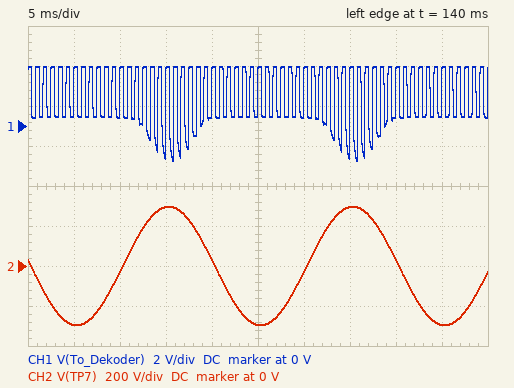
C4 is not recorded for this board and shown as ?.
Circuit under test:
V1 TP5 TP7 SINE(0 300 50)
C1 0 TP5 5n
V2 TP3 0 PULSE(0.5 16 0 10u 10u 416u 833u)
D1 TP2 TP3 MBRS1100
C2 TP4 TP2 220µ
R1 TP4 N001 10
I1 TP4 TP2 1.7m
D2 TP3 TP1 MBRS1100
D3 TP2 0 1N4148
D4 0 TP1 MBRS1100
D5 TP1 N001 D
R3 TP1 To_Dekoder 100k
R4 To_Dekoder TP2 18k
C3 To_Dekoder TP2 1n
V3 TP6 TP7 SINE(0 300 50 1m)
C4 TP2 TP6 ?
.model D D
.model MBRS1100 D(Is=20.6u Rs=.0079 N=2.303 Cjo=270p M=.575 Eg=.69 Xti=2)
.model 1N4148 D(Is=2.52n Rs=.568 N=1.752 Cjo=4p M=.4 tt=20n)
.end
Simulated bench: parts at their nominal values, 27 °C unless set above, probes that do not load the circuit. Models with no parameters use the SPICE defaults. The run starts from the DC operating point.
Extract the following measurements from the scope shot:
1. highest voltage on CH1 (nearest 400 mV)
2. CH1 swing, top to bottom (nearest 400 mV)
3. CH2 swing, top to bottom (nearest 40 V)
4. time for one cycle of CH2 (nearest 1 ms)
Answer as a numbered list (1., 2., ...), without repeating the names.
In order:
1. 2.8 V
2. 4.8 V
3. 600 V
4. 20 ms
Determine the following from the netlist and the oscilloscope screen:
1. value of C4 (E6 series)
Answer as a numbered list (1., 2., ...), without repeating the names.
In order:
1. 2.2 nF
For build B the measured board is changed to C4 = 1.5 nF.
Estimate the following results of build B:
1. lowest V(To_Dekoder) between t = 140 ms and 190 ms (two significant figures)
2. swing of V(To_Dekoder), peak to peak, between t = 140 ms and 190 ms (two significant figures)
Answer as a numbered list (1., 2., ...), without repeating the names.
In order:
1. -850 mV
2. 3.8 V
